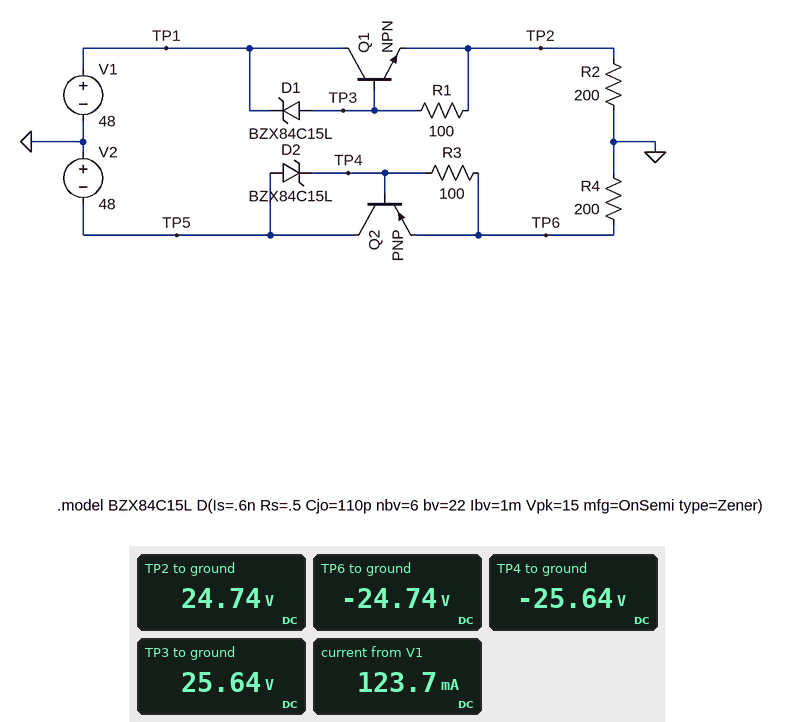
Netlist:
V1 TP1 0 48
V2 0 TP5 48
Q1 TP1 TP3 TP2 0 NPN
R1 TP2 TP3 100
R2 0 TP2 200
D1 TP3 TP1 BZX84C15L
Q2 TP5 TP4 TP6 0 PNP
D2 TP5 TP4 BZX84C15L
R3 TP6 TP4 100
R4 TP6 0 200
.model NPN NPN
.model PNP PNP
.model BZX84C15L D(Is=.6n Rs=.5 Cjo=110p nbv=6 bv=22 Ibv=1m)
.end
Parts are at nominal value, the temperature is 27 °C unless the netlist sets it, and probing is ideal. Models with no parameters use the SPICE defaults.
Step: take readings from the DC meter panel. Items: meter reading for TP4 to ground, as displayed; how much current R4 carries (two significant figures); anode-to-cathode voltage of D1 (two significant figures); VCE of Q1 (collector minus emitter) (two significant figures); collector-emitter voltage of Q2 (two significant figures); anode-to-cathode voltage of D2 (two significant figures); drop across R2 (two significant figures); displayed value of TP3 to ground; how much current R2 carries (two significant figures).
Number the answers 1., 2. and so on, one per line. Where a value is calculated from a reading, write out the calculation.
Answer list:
1. -25.64 V
2. (0 V - (-24.74 V)) / 200 Ω = 120 mA
3. 25.64 V - 48 V = -22 V
4. 48 V - 24.74 V = 23 V
5. -48 V - (-24.74 V) = -23 V
6. -48 V - (-25.64 V) = -22 V
7. 24.74 V = 25 V
8. 25.64 V
9. (24.74 V) / 200 Ω = 120 mA
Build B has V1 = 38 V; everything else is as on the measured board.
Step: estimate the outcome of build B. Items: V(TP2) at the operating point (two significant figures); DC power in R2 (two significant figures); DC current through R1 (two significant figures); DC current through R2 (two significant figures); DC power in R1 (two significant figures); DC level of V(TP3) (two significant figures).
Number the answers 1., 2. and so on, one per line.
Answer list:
1. 15 V
2. 1.1 W
3. 8.8 mA
4. 74 mA
5. 7.8 mW
6. 16 V
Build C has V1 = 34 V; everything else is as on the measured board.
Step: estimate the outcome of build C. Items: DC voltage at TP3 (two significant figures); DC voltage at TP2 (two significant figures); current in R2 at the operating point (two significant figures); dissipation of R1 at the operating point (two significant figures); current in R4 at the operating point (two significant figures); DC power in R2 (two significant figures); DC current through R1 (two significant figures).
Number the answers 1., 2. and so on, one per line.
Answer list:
1. 12 V
2. 11 V
3. 54 mA
4. 7.6 mW
5. 120 mA
6. 580 mW
7. 8.7 mA
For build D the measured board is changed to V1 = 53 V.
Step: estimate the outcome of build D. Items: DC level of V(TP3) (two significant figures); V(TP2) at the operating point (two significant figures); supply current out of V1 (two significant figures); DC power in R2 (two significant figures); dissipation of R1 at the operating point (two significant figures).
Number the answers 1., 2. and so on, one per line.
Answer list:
1. 31 V
2. 30 V
3. 150 mA
4. 4.4 W
5. 8.1 mW
